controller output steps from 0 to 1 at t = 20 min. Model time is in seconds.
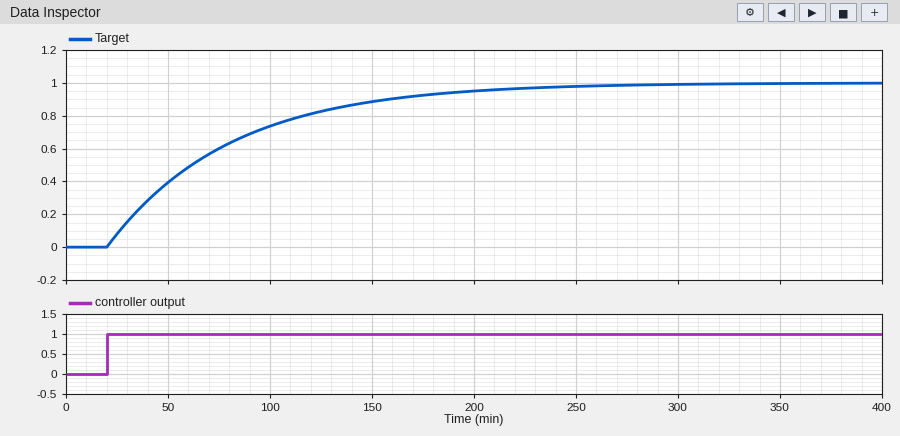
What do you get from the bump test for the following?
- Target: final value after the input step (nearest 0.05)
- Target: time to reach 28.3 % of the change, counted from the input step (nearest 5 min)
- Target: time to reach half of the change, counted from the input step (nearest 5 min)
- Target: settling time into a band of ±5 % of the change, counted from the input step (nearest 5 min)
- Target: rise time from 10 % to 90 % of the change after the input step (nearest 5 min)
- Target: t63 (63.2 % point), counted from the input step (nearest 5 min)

1.00
20 min
40 min
180 min
130 min
60 min
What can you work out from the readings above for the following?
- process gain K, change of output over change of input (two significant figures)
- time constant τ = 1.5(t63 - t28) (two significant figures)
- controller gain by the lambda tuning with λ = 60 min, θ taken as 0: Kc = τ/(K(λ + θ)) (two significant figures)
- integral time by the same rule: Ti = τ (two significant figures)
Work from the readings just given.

1.0
60 min
1.0
60 min
